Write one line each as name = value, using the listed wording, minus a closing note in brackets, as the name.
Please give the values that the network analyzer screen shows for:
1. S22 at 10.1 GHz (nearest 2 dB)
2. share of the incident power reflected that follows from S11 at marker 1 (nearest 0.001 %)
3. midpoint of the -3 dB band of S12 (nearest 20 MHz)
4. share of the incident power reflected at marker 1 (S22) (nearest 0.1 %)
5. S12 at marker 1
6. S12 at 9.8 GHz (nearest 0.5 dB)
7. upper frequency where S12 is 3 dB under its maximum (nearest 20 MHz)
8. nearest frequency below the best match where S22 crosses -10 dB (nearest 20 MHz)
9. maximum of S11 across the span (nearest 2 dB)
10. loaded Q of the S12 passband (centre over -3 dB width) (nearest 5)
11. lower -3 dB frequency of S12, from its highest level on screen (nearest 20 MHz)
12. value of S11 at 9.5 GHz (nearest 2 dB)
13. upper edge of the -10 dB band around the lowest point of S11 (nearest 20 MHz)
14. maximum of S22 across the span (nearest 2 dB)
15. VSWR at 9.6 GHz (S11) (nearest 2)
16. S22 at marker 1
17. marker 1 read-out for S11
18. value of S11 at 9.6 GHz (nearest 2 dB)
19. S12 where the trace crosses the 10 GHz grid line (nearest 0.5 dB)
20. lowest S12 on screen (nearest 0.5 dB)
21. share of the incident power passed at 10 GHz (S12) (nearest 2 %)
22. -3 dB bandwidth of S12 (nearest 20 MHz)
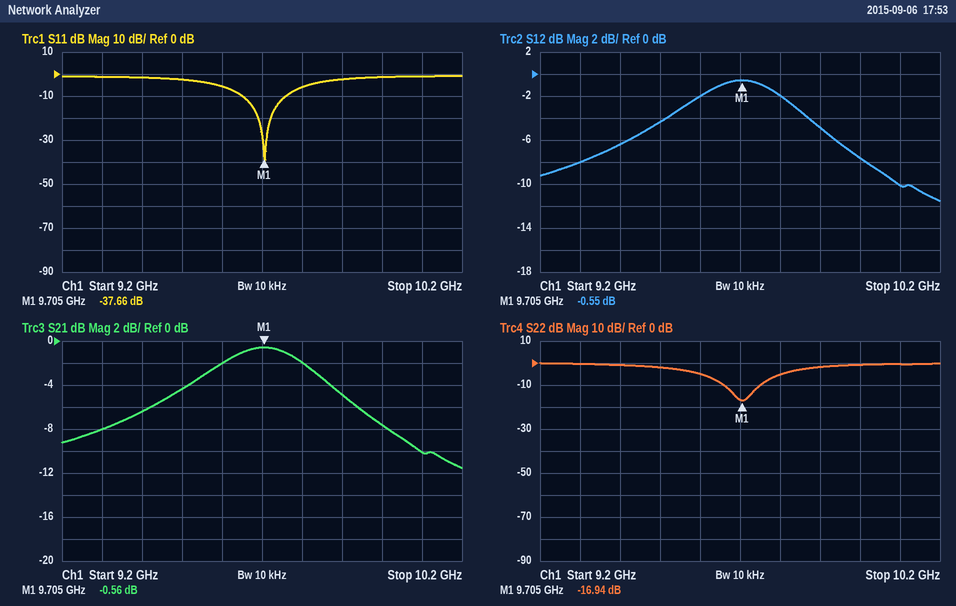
S22 at 10.1 GHz = 0 dB
share of the incident power reflected that follows from S11 at marker 1 = 0.017 %
midpoint of the -3 dB band of S12 = 9.70 GHz
share of the incident power reflected at marker 1 (S22) = 2.0 %
S12 at marker 1 = -0.55 dB
S12 at 9.8 GHz = -2.0 dB
upper frequency where S12 is 3 dB under its maximum = 9.86 GHz
nearest frequency below the best match where S22 crosses -10 dB = 9.66 GHz
maximum of S11 across the span = 0 dB
loaded Q of the S12 passband (centre over -3 dB width) = 30
lower -3 dB frequency of S12, from its highest level on screen = 9.54 GHz
value of S11 at 9.5 GHz = -2 dB
upper edge of the -10 dB band around the lowest point of S11 = 9.76 GHz
maximum of S22 across the span = 0 dB
VSWR at 9.6 GHz (S11) = 4
S22 at marker 1 = -16.94 dB
marker 1 read-out for S11 = -37.66 dB
value of S11 at 9.6 GHz = -6 dB
S12 where the trace crosses the 10 GHz grid line = -7.5 dB
lowest S12 on screen = -11.5 dB
share of the incident power passed at 10 GHz (S12) = 18 %
-3 dB bandwidth of S12 = 320 MHz
